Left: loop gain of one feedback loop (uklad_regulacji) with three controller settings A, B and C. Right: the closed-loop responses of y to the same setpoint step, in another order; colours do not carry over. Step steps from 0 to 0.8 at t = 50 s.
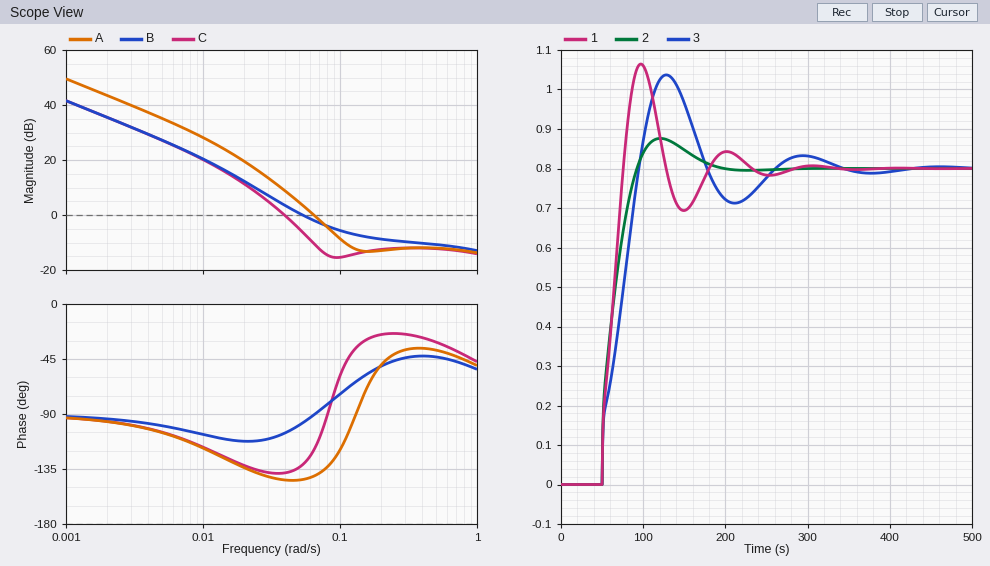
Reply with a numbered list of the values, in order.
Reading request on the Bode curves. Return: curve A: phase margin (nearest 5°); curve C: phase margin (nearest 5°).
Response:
1. 40°
2. 40°
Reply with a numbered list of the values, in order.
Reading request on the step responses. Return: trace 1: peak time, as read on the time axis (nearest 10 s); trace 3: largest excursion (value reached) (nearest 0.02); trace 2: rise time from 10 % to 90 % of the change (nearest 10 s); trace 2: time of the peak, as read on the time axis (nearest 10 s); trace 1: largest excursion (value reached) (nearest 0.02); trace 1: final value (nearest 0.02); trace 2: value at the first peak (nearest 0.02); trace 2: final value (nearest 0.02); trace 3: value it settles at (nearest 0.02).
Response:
1. 100 s
2. 1.04
3. 30 s
4. 120 s
5. 1.06
6. 0.80
7. 0.88
8. 0.80
9. 0.80
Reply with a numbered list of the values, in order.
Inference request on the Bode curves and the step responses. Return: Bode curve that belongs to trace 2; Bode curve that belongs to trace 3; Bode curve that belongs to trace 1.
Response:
1. B
2. C
3. A
